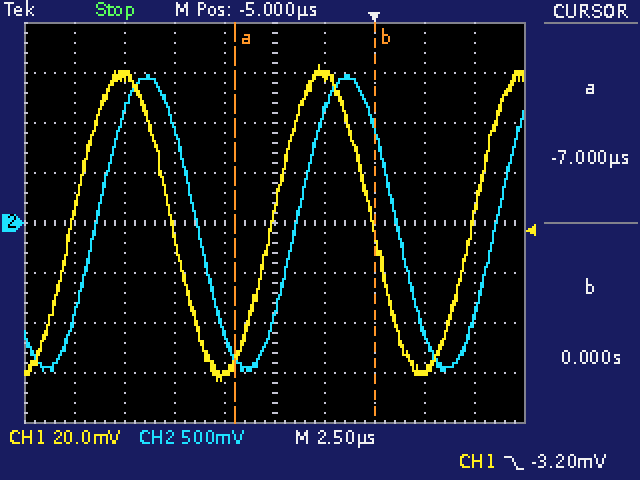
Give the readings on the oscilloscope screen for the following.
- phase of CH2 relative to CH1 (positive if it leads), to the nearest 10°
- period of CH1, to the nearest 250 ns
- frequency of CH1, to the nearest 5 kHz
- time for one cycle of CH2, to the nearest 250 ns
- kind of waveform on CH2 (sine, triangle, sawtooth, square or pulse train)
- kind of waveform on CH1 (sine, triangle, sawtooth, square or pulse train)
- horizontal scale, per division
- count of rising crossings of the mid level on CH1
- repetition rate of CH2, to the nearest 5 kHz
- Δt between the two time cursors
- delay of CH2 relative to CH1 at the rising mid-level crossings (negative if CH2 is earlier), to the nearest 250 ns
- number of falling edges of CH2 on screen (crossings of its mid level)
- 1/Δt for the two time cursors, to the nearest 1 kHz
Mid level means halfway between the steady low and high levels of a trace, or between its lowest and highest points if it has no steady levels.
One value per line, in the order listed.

-40°
10.00 µs
100 kHz
10.00 µs
sine
sine
2.5 µs
3
100 kHz
7.00 µs
+1.25 µs
2
143 kHz
